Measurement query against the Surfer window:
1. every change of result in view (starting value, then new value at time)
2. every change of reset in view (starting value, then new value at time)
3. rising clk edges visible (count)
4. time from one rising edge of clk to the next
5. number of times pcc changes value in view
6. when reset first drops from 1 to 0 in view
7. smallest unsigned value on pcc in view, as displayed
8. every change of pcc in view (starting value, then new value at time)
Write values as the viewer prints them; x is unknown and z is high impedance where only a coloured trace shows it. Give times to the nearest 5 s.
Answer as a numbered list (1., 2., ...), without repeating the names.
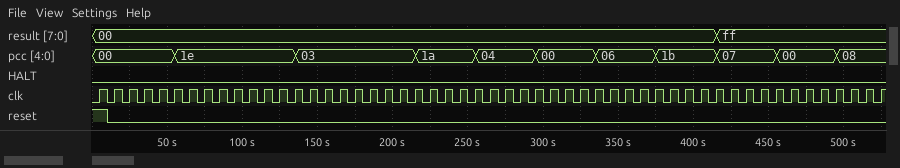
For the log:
1. 00, ff at 415 s
2. 1, 0 at 10 s
3. 53
4. 10 s
5. 10
6. 10 s
7. 00
8. 00, 1e at 55 s, 03 at 135 s, 1a at 215 s, 04 at 255 s, 00 at 295 s, 06 at 335 s, 1b at 375 s, 07 at 415 s, 00 at 455 s, 08 at 495 s
